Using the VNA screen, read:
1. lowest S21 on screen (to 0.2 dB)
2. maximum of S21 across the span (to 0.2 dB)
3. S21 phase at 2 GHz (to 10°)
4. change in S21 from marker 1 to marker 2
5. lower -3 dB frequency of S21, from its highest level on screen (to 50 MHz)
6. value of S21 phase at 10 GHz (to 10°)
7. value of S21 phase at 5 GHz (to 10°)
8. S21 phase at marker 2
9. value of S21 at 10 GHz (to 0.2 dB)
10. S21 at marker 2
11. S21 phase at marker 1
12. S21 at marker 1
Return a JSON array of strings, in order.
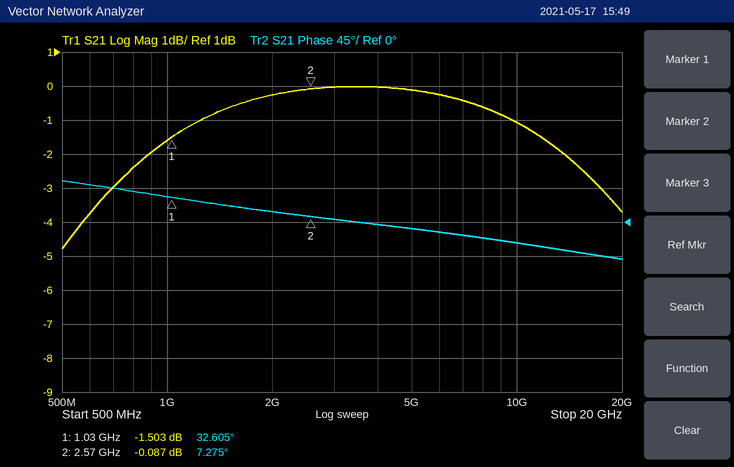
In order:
["-4.8 dB", "0.0 dB", "10°", "1.416 dB", "700 MHz", "-30°", "-10°", "7.275°", "-1.0 dB", "-0.087 dB", "32.605°", "-1.503 dB"]
